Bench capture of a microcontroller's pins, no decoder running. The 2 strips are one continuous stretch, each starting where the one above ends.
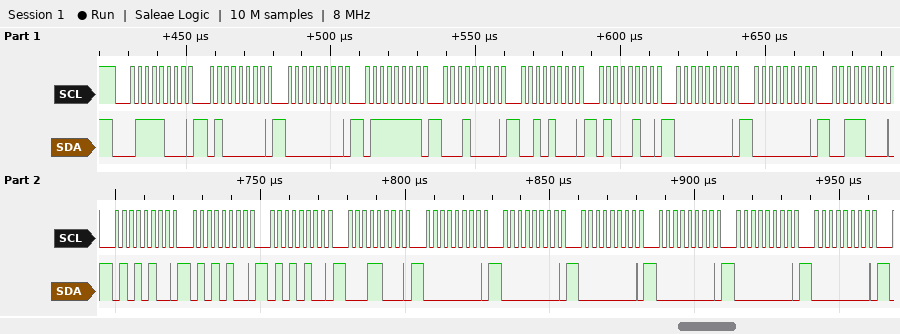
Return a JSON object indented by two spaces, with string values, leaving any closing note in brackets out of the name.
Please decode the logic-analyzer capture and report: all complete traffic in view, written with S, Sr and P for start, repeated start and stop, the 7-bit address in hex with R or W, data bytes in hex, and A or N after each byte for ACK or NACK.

{
  "all complete traffic in view, written with S, Sr and P for start, repeated start and stop, the 7-bit address in hex with R or W, data bytes in hex, and A or N after each byte for ACK or NACK": "S 3CW A 40 A 00 A 7F A 10 A 28 A 44 A 00 A 00 A 38 A 54 A 54 A 54 A 18 A 00 A 00 A 00 A 00 A 00 A 00 A"
}
